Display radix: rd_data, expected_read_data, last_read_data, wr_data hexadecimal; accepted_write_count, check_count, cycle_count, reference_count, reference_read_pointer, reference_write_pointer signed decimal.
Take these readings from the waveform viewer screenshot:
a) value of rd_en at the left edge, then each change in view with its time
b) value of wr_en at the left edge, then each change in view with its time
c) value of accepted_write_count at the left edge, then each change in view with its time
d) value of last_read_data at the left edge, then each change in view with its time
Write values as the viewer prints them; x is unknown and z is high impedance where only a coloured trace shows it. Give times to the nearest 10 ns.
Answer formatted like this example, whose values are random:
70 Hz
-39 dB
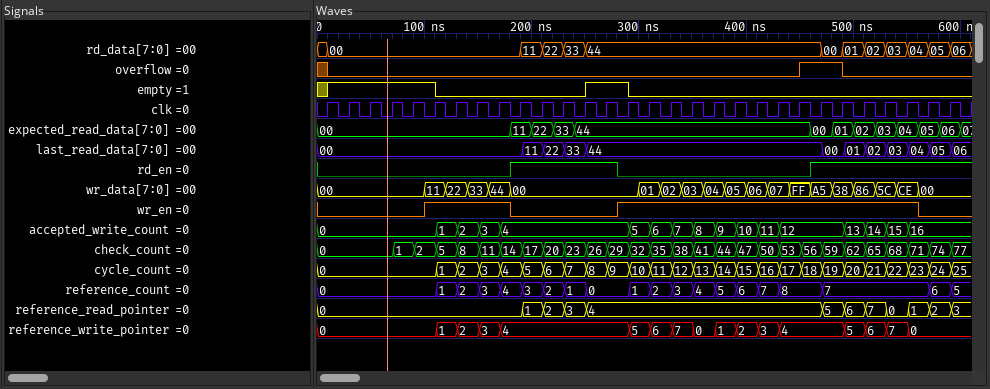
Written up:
0, 1 at 180 ns, 0 at 280 ns, 1 at 460 ns
0, 1 at 100 ns, 0 at 180 ns, 1 at 280 ns, 0 at 560 ns
0, 1 at 110 ns, 2 at 130 ns, 3 at 150 ns, 4 at 170 ns, 5 at 290 ns, 6 at 310 ns, 7 at 330 ns, 8 at 350 ns, 9 at 370 ns, 10 at 390 ns, 11 at 410 ns, 12 at 430 ns, 13 at 490 ns, 14 at 510 ns, 15 at 530 ns, 16 at 550 ns
00, 11 at 190 ns, 22 at 210 ns, 33 at 230 ns, 44 at 250 ns, 00 at 470 ns, 01 at 490 ns, 02 at 510 ns, 03 at 530 ns, 04 at 550 ns, 05 at 570 ns, 06 at 590 ns
